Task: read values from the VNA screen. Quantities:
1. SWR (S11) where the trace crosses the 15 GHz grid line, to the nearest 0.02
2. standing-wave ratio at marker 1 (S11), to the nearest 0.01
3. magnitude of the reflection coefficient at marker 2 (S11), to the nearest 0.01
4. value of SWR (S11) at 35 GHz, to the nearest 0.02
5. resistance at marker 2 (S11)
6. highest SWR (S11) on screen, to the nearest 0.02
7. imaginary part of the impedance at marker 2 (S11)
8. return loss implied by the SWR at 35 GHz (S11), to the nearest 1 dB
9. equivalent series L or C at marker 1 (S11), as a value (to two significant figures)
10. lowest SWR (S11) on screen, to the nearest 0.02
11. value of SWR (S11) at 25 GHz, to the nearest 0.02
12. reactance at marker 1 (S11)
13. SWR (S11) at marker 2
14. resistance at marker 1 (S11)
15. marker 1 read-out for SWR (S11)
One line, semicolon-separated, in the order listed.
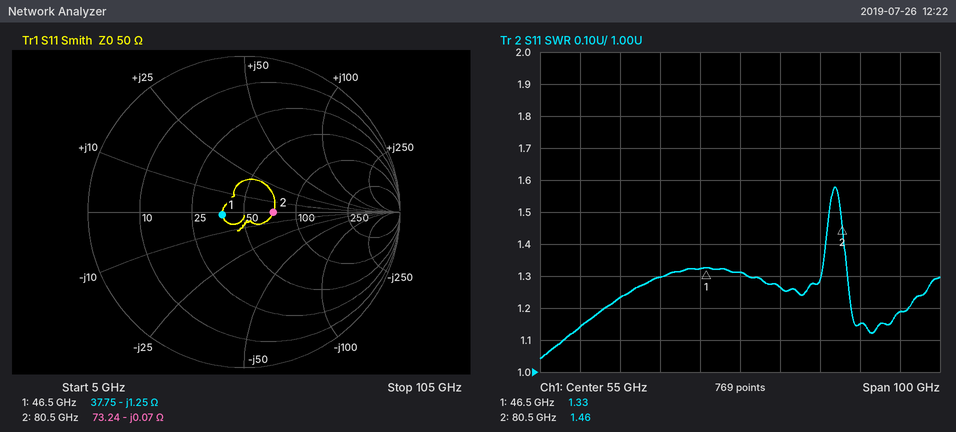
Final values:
1.14; 1.33; 0.19; 1.30; 73.24 Ω; 1.58; -0.07 Ω; 18 dB; 2.7 pF; 1.04; 1.24; -1.25 Ω; 1.46; 37.75 Ω; 1.33
